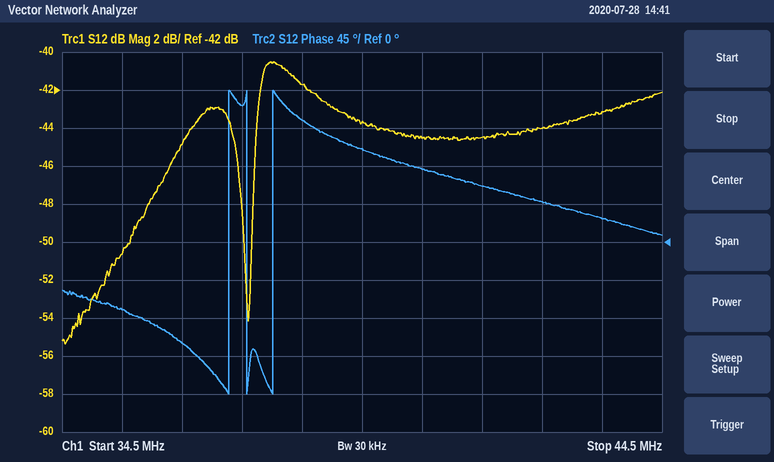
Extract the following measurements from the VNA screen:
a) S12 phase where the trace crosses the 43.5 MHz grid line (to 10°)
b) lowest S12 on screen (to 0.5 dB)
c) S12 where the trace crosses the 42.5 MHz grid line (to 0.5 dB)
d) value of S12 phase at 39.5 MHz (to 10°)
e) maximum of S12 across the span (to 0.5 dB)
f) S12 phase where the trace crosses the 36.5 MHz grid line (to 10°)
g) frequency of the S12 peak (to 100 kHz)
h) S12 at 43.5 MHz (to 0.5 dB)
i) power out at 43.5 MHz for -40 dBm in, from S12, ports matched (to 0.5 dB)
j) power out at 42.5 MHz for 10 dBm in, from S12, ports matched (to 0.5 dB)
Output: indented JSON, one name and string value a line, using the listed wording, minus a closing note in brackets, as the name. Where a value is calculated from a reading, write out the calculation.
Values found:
{
  "S12 phase where the trace crosses the 43.5 MHz grid line": "30°",
  "lowest S12 on screen": "-55.5 dB",
  "S12 where the trace crosses the 42.5 MHz grid line": "-44.0 dB",
  "value of S12 phase at 39.5 MHz": "110°",
  "maximum of S12 across the span": "-40.5 dB",
  "S12 phase where the trace crosses the 36.5 MHz grid line": "-120°",
  "frequency of the S12 peak": "38.0 MHz",
  "S12 at 43.5 MHz": "-43.0 dB",
  "power out at 43.5 MHz for -40 dBm in, from S12, ports matched": "-40 dBm + (-43.0 dB) = -83.0 dBm",
  "power out at 42.5 MHz for 10 dBm in, from S12, ports matched": "10 dBm + (-44.0 dB) = -34.0 dBm"
}
